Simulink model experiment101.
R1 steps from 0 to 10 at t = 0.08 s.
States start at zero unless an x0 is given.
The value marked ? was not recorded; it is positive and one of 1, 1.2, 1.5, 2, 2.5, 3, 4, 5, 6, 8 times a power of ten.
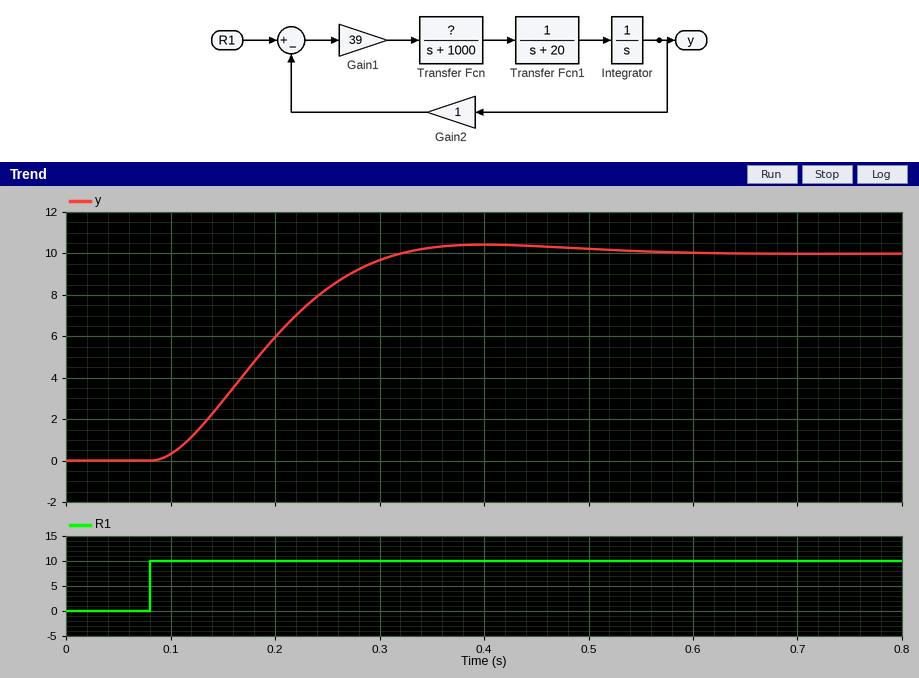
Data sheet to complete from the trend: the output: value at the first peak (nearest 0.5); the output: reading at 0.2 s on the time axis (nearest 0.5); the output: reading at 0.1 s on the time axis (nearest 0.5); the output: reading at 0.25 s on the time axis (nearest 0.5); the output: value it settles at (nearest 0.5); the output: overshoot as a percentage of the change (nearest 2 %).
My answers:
10.5
6.0
0.5
8.5
10.0
4 %
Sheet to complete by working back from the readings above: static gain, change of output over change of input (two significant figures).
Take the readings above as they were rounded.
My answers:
1.0
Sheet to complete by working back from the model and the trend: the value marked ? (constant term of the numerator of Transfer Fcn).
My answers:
5000
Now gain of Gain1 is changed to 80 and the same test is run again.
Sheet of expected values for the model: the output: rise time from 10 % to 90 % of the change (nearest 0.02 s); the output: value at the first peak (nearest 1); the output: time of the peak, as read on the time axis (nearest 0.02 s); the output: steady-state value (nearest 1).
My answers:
0.08 s
12
0.26 s
10
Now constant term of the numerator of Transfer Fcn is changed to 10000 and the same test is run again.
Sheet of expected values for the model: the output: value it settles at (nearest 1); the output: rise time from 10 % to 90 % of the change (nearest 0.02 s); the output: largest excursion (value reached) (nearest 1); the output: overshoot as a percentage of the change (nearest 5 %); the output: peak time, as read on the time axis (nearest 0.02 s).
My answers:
10
0.08 s
12
15 %
0.26 s
